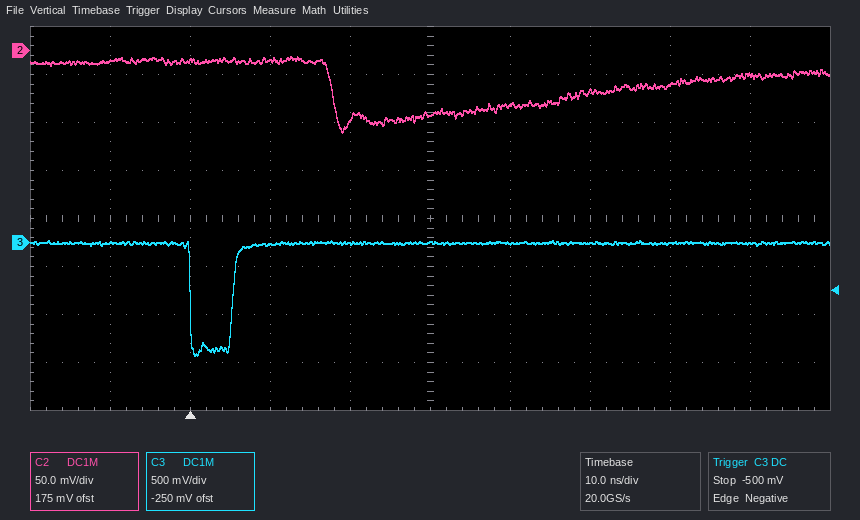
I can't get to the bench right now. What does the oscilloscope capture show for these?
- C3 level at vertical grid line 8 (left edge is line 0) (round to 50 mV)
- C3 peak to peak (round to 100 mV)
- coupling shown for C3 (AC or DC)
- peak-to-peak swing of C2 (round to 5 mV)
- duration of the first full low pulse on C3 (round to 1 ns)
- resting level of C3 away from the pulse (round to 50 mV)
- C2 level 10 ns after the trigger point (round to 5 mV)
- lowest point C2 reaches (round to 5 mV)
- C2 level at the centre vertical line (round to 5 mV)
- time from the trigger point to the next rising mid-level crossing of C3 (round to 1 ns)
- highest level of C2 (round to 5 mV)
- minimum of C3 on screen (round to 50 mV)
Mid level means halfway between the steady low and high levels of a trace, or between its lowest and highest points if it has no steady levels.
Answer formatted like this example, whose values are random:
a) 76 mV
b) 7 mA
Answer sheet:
a) 0 mV
b) 1.20 V
c) DC
d) 80 mV
e) 5 ns
f) 0 mV
g) -10 mV
h) -85 mV
i) -65 mV
j) 5 ns
k) -5 mV
l) -1.20 V
